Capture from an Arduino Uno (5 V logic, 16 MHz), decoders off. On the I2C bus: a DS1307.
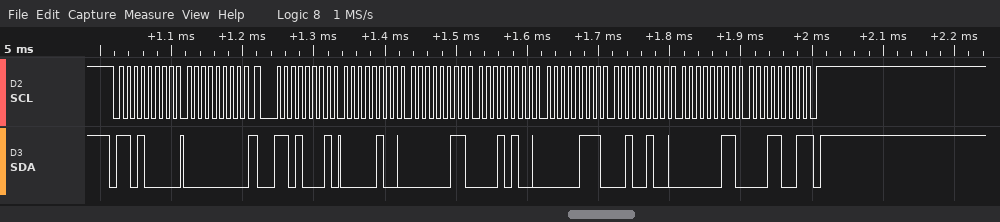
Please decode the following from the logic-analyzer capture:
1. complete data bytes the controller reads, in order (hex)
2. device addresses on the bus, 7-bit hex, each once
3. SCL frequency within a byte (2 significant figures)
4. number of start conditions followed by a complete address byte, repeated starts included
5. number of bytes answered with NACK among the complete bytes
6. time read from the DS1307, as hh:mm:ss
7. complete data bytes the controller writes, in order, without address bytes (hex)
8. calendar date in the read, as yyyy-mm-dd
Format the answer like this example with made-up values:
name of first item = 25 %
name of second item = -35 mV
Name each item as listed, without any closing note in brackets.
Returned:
complete data bytes the controller reads, in order = 04 03 14 07 24 03 19
device addresses on the bus, 7-bit hex, each once = 0x68
SCL frequency within a byte = 100 kHz
number of start conditions followed by a complete address byte, repeated starts included = 2
number of bytes answered with NACK among the complete bytes = 1
time read from the DS1307, as hh:mm:ss = 14:03:04
complete data bytes the controller writes, in order, without address bytes = 00
calendar date in the read, as yyyy-mm-dd = 2019-03-24
